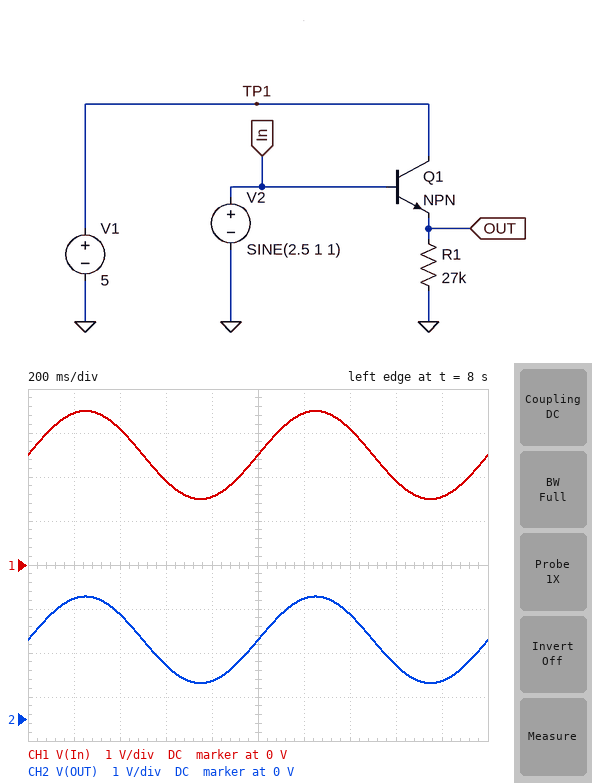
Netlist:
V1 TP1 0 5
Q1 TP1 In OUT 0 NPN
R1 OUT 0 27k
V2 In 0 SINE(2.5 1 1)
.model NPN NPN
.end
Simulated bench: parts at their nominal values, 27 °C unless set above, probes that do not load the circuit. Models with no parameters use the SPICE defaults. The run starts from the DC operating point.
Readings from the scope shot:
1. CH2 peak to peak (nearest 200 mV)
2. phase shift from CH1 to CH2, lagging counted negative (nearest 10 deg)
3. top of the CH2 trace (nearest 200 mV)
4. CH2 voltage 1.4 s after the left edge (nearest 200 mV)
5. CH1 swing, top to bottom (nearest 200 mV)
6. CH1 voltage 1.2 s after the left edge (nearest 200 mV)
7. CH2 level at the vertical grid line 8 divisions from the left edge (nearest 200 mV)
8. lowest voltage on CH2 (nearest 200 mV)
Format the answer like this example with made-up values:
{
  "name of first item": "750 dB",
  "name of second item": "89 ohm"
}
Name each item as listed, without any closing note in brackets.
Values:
{
  "CH2 peak to peak": "2.0 V",
  "phase shift from CH1 to CH2, lagging counted negative": "0 deg",
  "top of the CH2 trace": "2.8 V",
  "CH2 voltage 1.4 s after the left edge": "2.4 V",
  "CH1 swing, top to bottom": "2.0 V",
  "CH1 voltage 1.2 s after the left edge": "3.4 V",
  "CH2 level at the vertical grid line 8 divisions from the left edge": "1.2 V",
  "lowest voltage on CH2": "800 mV"
}
